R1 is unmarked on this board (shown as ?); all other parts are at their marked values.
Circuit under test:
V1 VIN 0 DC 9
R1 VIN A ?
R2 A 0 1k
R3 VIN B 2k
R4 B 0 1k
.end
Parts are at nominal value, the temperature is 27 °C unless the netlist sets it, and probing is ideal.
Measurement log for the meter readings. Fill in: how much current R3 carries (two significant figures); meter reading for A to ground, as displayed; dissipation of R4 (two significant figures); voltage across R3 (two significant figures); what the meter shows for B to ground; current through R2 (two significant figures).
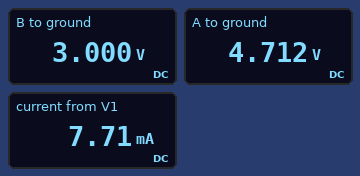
3.0 mA
4.712 V
9.0 mW
6.0 V
3.000 V
4.7 mA
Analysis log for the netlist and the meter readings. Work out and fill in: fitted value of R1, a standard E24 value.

910 Ω
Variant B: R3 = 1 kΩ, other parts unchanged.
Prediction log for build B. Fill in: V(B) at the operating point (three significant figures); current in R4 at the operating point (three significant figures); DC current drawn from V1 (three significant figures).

4.50 V
4.50 mA
9.21 mA
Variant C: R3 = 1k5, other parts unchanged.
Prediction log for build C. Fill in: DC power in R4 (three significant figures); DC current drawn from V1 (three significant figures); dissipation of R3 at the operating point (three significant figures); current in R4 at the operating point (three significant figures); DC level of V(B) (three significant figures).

13.0 mW
8.31 mA
19.4 mW
3.60 mA
3.60 V
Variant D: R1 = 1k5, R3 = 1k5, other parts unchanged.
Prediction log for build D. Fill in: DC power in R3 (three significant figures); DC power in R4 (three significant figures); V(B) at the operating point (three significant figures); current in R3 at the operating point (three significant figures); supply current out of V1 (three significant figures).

19.4 mW
13.0 mW
3.60 V
3.60 mA
7.20 mA
